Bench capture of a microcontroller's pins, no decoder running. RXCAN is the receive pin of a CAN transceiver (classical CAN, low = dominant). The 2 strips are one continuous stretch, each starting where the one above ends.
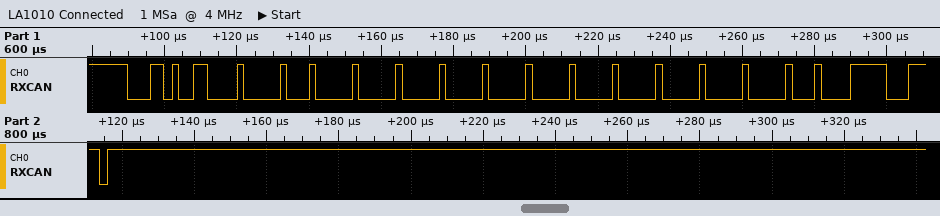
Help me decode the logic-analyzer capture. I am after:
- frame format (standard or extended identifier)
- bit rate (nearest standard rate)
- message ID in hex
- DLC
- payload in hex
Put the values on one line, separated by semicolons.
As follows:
standard; 500 kbit/s; 0x1A6; 8; 04 00 00 00 00 00 00 00
